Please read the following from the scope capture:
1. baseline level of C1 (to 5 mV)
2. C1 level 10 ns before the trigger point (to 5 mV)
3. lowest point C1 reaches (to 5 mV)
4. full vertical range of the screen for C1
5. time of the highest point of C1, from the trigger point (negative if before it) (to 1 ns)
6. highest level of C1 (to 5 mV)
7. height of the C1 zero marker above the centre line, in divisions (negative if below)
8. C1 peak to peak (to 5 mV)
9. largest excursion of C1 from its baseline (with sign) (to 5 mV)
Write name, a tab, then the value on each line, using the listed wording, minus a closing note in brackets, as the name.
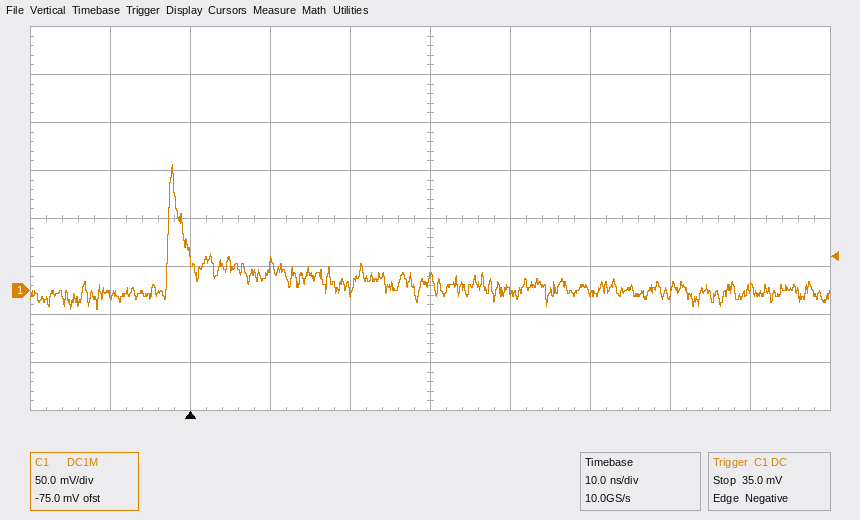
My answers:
baseline level of C1	0 mV
C1 level 10 ns before the trigger point	-5 mV
lowest point C1 reaches	-20 mV
full vertical range of the screen for C1	400 mV
time of the highest point of C1, from the trigger point (negative if before it)	-2 ns
highest level of C1	130 mV
height of the C1 zero marker above the centre line, in divisions	-1.5 div
C1 peak to peak	150 mV
largest excursion of C1 from its baseline (with sign)	+130 mV
